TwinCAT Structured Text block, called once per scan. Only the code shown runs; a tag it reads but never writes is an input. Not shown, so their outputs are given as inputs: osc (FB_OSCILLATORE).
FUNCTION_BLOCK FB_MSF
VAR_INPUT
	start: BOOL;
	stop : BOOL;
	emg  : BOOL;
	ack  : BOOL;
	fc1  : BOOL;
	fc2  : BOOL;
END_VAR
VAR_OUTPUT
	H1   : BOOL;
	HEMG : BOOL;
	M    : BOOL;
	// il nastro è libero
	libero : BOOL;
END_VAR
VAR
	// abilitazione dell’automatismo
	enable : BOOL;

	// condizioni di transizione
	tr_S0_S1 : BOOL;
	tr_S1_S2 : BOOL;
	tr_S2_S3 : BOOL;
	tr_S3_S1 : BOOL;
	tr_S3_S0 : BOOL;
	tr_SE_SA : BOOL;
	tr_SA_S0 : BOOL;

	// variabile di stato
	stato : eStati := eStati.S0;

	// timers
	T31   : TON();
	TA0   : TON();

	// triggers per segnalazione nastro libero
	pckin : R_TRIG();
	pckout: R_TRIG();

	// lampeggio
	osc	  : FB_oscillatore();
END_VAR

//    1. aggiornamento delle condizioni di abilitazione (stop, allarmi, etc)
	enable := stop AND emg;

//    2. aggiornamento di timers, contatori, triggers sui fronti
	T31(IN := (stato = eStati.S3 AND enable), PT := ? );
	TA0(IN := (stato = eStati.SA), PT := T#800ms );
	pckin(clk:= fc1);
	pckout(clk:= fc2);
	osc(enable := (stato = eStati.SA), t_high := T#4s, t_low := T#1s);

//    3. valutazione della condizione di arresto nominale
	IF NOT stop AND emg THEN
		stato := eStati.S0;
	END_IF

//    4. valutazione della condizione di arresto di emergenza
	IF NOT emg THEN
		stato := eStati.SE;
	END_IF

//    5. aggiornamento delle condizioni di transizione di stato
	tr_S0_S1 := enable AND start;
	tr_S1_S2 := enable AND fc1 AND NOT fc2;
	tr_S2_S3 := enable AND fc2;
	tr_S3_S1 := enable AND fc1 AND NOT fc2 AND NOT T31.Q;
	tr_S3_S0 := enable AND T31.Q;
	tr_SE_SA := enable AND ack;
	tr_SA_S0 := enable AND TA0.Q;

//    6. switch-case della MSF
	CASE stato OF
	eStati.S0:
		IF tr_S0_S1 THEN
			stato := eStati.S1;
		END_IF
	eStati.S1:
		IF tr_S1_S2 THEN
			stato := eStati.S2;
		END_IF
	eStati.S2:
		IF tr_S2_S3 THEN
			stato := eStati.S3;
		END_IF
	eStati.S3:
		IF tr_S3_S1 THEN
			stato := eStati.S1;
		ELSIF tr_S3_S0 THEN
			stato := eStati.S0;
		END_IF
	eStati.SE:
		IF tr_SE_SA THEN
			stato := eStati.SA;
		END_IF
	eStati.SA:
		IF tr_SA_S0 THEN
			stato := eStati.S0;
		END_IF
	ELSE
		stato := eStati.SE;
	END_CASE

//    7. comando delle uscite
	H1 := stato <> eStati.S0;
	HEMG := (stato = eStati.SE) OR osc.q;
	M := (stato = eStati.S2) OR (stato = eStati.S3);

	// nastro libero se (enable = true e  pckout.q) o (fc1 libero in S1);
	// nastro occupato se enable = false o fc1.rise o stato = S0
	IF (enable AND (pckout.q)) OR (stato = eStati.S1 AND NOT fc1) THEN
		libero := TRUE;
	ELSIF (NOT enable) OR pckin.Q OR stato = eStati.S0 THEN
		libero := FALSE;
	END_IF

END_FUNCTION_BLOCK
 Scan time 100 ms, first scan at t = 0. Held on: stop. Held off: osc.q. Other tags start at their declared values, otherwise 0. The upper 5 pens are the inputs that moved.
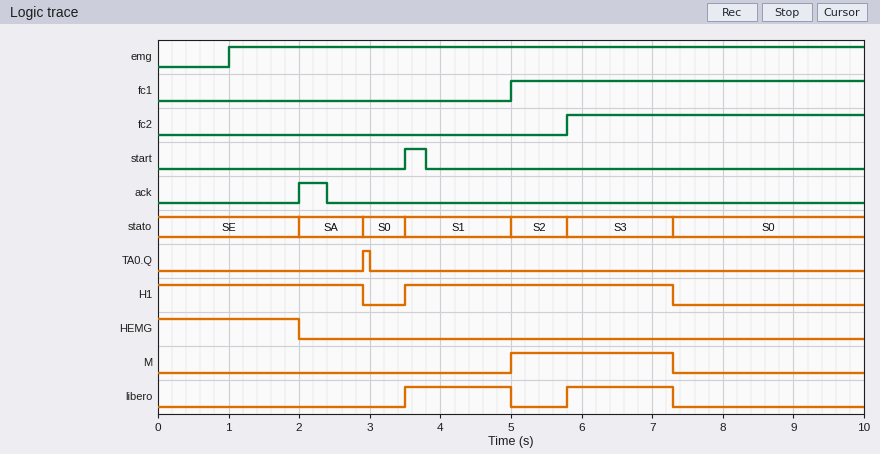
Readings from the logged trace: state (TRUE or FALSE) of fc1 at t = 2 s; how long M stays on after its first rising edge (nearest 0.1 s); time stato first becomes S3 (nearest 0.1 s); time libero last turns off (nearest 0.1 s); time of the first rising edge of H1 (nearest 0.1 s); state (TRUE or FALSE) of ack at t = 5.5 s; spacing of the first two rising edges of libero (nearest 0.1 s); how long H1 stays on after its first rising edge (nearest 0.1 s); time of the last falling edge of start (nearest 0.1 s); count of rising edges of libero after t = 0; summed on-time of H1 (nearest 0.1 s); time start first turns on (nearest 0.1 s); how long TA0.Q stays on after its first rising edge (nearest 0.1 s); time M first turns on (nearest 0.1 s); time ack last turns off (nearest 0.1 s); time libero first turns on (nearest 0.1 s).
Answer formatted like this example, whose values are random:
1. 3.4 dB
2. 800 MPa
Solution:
1. FALSE
2. 2.3 s
3. 5.8 s
4. 7.3 s
5. 3.5 s
6. FALSE
7. 2.3 s
8. 3.8 s
9. 3.8 s
10. 2
11. 6.7 s
12. 3.5 s
13. 0.1 s
14. 5.0 s
15. 2.4 s
16. 3.5 s
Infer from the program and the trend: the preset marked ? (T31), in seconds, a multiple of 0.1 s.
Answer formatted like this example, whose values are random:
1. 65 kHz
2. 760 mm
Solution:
1. 1.4 s
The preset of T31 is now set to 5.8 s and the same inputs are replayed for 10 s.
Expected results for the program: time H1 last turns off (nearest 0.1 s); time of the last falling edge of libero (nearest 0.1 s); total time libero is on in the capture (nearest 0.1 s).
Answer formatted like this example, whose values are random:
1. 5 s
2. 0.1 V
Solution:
1. 2.9 s
2. 5.0 s
3. 5.7 s
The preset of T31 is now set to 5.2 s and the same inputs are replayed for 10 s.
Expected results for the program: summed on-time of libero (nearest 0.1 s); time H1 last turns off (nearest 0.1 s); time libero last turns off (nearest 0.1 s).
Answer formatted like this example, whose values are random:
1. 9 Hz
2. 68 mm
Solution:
1. 5.7 s
2. 2.9 s
3. 5.0 s
